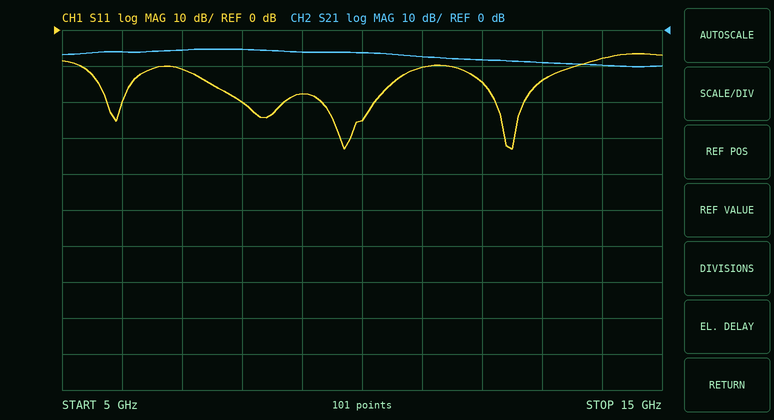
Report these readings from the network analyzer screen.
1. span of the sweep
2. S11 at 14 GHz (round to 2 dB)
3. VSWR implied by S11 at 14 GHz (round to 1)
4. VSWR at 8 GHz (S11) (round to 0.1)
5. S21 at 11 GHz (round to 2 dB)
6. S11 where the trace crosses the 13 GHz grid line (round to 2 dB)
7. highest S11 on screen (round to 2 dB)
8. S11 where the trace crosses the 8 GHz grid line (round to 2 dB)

10 GHz
-8 dB
2
1.2
-8 dB
-14 dB
-6 dB
-20 dB
